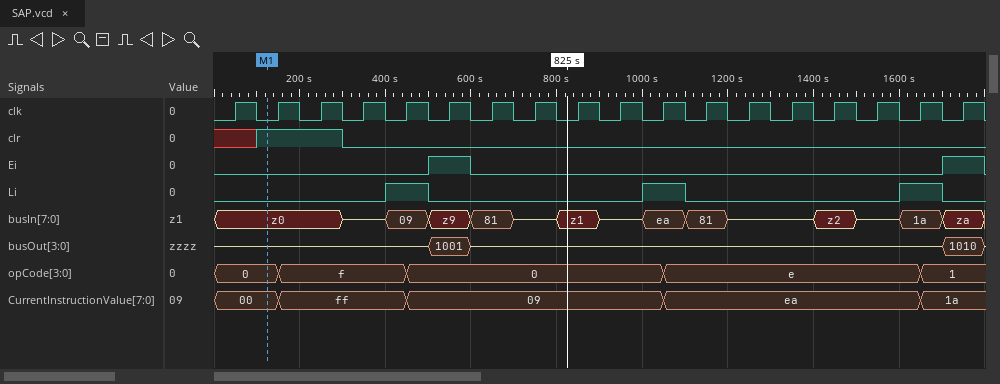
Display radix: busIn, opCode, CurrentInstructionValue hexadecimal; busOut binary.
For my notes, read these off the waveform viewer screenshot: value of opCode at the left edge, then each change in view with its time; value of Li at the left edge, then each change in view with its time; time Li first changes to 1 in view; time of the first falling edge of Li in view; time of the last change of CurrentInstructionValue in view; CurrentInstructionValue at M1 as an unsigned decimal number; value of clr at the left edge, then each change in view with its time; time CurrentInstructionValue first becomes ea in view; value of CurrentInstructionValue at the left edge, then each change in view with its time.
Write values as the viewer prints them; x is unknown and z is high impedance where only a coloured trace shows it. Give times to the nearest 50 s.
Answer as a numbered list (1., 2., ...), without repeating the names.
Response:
1. 0, f at 150 s, 0 at 450 s, e at 1050 s, 1 at 1650 s
2. 0, 1 at 400 s, 0 at 500 s, 1 at 1000 s, 0 at 1100 s, 1 at 1600 s, 0 at 1700 s
3. 400 s
4. 500 s
5. 1650 s
6. 0
7. x, 1 at 100 s, 0 at 300 s
8. 1050 s
9. 00, ff at 150 s, 09 at 450 s, ea at 1050 s, 1a at 1650 s
